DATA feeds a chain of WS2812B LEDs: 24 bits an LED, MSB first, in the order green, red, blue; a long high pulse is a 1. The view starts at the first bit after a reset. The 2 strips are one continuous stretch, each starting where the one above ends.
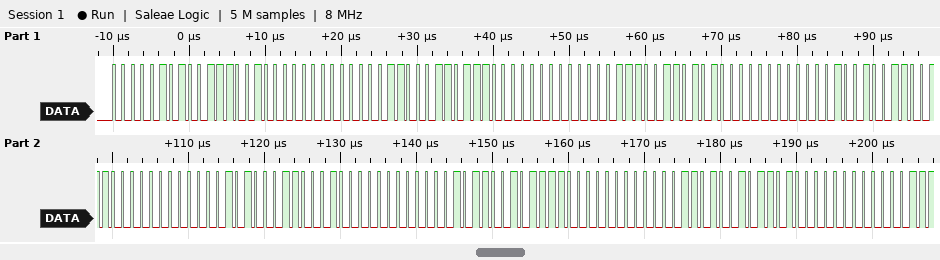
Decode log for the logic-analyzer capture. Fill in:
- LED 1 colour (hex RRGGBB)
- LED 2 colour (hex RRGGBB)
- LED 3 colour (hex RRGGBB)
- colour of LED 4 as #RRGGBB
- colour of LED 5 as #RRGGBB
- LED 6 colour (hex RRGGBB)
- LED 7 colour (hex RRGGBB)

#390500
#370600
#350700
#330900
#310A00
#2F0B00
#2D0D00
